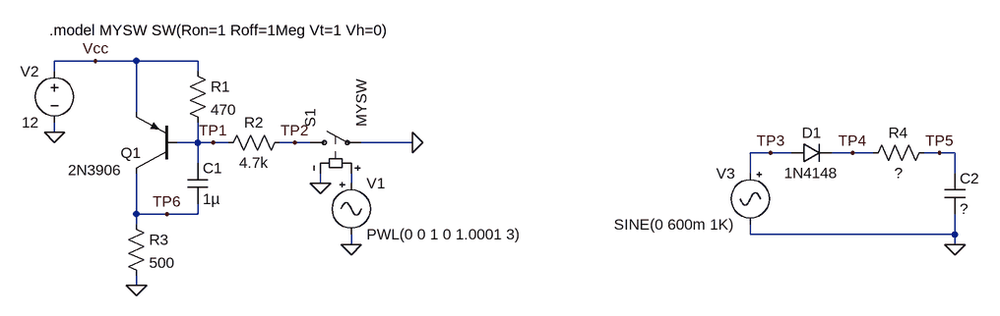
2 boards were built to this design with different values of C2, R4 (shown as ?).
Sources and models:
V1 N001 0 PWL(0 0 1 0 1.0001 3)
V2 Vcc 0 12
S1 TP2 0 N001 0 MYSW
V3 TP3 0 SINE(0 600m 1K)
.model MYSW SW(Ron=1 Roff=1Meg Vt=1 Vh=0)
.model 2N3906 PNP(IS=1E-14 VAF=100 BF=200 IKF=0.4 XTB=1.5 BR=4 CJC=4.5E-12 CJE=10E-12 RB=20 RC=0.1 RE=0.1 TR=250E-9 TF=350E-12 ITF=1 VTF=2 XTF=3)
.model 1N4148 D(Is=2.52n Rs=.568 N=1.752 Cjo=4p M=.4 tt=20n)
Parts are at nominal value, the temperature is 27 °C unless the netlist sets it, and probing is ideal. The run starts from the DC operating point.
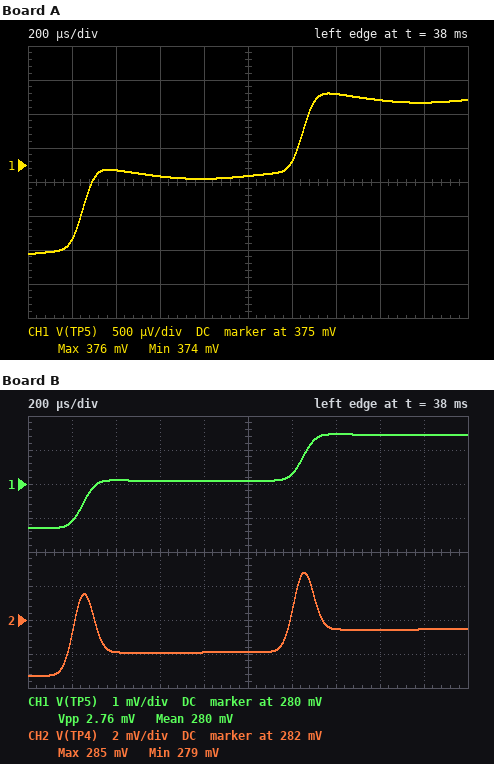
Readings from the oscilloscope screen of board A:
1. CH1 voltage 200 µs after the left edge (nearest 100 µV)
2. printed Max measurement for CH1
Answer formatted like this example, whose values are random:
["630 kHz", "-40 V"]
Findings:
["373.9 mV", "376 mV"]
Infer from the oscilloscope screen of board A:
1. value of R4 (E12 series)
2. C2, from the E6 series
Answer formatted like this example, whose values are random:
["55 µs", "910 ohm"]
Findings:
["330 Ω", "33 nF"]
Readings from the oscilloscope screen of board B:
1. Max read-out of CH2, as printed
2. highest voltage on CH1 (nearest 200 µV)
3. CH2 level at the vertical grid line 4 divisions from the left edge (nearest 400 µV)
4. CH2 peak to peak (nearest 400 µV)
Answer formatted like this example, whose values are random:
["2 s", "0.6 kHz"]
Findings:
["285 mV", "281.4 mV", "280.0 mV", "6.0 mV"]
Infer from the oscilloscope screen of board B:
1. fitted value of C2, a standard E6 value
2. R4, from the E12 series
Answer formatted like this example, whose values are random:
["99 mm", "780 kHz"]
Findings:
["220 nF", "1.5 kΩ"]
